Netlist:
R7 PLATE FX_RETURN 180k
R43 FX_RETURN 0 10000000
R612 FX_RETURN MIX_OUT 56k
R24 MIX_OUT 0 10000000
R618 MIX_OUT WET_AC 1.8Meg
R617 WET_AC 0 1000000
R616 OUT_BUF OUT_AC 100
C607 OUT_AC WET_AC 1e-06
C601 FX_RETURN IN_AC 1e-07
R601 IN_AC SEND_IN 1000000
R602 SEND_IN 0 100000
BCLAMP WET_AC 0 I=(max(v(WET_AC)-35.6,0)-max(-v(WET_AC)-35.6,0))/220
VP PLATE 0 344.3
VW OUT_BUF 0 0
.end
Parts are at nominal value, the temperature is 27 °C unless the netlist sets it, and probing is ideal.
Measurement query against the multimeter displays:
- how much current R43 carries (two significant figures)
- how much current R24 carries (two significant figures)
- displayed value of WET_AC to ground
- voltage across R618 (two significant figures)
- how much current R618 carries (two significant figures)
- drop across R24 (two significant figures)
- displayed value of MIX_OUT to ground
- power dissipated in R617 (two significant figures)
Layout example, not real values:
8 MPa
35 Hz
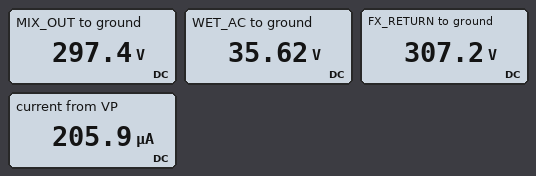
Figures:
31 µA
30 µA
35.62 V
260 V
150 µA
300 V
297.4 V
1.3 mW
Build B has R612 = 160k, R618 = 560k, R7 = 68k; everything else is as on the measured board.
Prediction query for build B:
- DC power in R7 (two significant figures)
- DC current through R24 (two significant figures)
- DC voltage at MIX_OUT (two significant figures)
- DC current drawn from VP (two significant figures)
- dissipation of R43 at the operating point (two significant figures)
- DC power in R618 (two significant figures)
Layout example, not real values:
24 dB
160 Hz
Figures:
13 mW
25 µA
250 V
440 µA
9.9 mW
82 mW
